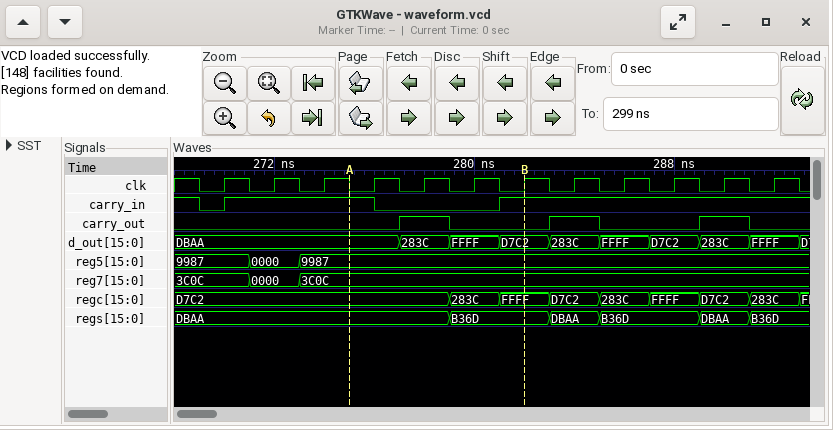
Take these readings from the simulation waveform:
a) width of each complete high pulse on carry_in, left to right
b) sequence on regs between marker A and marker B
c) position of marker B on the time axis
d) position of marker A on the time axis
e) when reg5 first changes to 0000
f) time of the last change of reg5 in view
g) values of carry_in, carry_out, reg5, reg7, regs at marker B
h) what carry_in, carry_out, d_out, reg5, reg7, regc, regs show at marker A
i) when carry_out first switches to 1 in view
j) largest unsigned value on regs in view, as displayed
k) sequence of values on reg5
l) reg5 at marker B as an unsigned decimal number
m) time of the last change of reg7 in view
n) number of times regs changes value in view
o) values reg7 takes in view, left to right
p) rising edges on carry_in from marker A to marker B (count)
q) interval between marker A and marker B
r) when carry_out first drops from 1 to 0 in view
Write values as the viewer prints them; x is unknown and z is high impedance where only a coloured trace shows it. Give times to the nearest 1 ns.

6 ns
DBAA, B36D
282 ns
275 ns
271 ns
273 ns
carry_in=1, carry_out=0, reg5=9987, reg7=3C0C, regs=B36D
carry_in=1, carry_out=0, d_out=DBAA, reg5=9987, reg7=3C0C, regc=D7C2, regs=DBAA
277 ns
DBAA
9987, 0000, 9987
39303
273 ns
5
3C0C, 0000, 3C0C
1
7 ns
279 ns
